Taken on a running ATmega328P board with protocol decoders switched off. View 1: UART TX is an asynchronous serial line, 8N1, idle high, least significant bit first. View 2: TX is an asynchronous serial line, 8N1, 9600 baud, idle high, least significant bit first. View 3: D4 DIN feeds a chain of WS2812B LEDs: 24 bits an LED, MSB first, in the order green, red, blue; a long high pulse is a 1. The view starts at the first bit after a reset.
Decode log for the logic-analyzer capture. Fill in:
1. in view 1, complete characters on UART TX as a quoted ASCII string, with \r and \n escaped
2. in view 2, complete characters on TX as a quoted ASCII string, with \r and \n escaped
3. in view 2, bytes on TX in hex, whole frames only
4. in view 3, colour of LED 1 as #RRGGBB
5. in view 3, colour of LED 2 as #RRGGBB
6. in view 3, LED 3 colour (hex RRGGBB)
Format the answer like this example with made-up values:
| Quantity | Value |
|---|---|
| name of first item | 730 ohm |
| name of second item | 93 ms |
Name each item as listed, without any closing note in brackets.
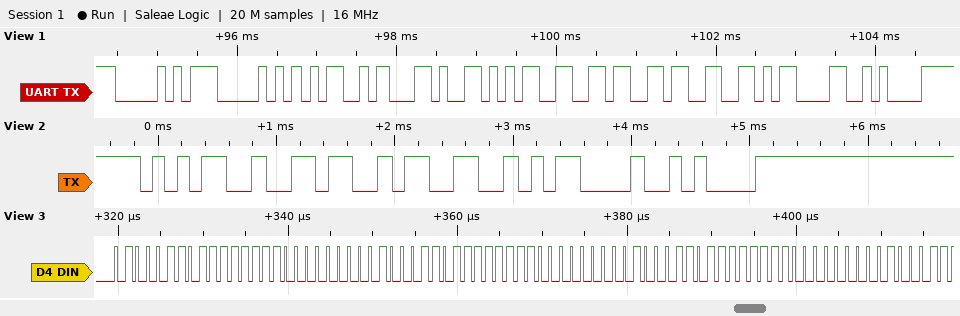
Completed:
| Quantity | Value |
|---|---|
| in view 1, complete characters on UART TX as a quoted ASCII string, with \r and \n escaped | "PPM,563\r\n" |
| in view 2, complete characters on TX as a quoted ASCII string, with \r and \n escaped | "563\r\n" |
| in view 2, bytes on TX in hex, whole frames only | 35 36 33 0D 0A |
| in view 3, colour of LED 1 as #RRGGBB | #FF4600 |
| in view 3, colour of LED 2 as #RRGGBB | #FF4600 |
| in view 3, LED 3 colour | #FF4600 |
